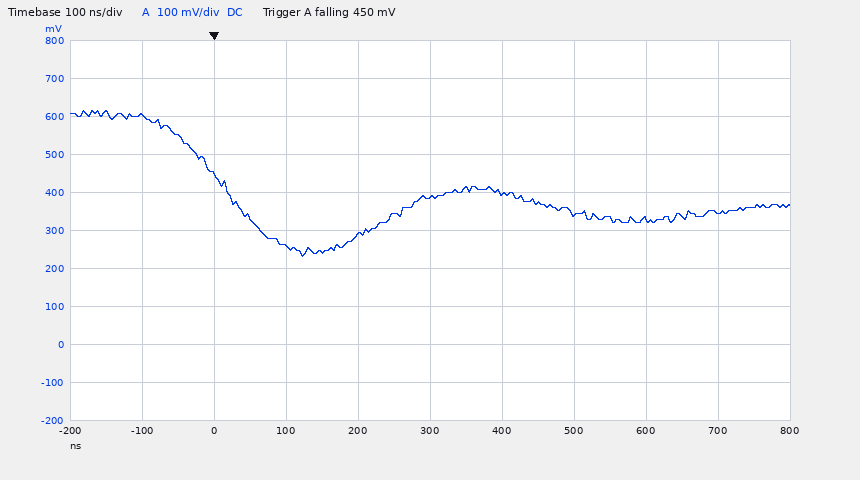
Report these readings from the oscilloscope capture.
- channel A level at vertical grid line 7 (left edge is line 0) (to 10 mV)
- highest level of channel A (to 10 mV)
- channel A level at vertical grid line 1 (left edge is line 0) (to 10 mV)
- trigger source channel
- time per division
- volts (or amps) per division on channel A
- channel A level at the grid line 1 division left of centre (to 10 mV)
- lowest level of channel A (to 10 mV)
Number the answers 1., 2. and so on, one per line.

1. 340 mV
2. 620 mV
3. 600 mV
4. channel A
5. 100 ns
6. 100 mV
7. 290 mV
8. 230 mV
